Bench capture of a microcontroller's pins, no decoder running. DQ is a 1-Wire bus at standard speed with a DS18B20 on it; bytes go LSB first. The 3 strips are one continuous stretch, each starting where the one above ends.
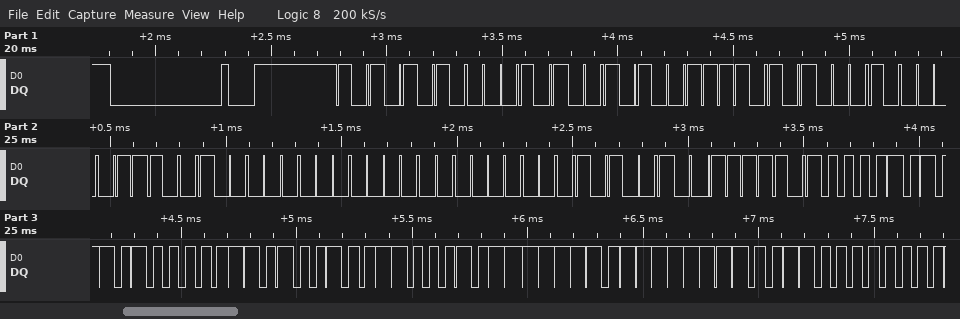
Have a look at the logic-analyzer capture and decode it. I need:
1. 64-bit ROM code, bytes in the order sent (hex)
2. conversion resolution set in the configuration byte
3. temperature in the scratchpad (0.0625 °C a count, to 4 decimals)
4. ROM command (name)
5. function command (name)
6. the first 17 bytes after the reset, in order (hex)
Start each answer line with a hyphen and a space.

- 28 E5 15 C1 09 00 00 4A
- 12 bits
- 85.0000 °C
- Match ROM
- Read Scratchpad
- 55 28 E5 15 C1 09 00 00 4A BE 50 05 4B 46 7F FF 0C
